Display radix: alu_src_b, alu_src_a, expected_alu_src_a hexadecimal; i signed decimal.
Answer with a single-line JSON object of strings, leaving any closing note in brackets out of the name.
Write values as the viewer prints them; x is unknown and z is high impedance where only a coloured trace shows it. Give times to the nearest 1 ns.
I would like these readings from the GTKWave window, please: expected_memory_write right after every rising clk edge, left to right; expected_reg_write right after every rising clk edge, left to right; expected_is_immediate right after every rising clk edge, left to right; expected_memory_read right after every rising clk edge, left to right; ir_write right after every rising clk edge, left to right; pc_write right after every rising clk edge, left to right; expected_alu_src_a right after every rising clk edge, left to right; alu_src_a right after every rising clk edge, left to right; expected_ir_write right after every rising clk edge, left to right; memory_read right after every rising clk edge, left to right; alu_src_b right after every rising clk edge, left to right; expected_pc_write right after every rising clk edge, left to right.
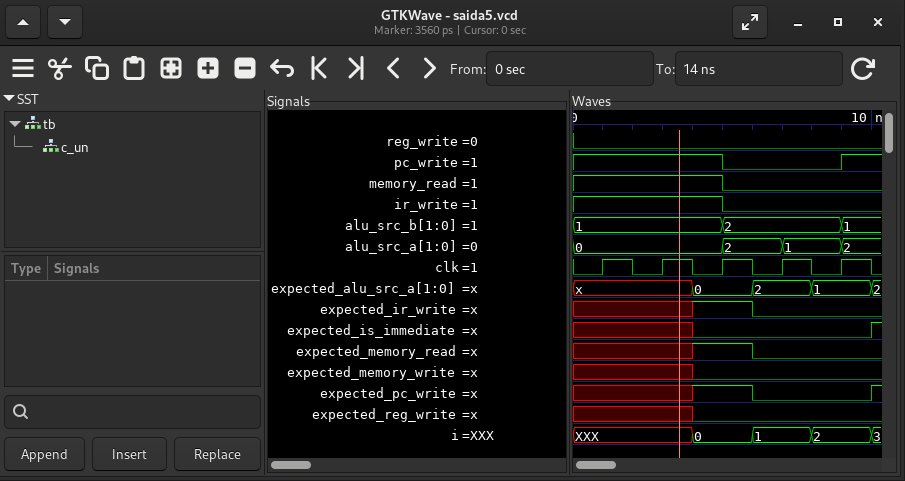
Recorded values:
{"expected_memory_write right after every rising clk edge, left to right": "x x 0 0 0", "expected_reg_write right after every rising clk edge, left to right": "x x 0 0 0", "expected_is_immediate right after every rising clk edge, left to right": "x x 0 0 0", "expected_memory_read right after every rising clk edge, left to right": "x x 1 0 0", "ir_write right after every rising clk edge, left to right": "1 1 0 0 0", "pc_write right after every rising clk edge, left to right": "1 1 0 0 1", "expected_alu_src_a right after every rising clk edge, left to right": "x, x, 0, 2, 1", "alu_src_a right after every rising clk edge, left to right": "0, 0, 2, 1, 2", "expected_ir_write right after every rising clk edge, left to right": "x x 1 0 0", "memory_read right after every rising clk edge, left to right": "1 1 0 0 0", "alu_src_b right after every rising clk edge, left to right": "1, 1, 2, 2, 1", "expected_pc_write right after every rising clk edge, left to right": "x x 1 0 0"}
